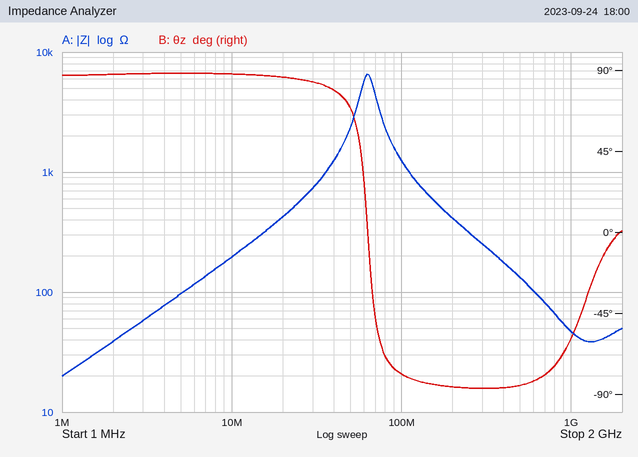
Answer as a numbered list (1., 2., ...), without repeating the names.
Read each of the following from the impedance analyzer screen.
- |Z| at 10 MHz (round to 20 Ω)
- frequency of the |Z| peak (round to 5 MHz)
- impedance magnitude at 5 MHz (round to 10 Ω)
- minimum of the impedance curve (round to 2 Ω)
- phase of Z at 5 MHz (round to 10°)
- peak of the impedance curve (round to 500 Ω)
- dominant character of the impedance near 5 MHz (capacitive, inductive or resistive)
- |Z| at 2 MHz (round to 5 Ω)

1. 200 Ω
2. 65 MHz
3. 100 Ω
4. 20 Ω
5. 90°
6. 6.5 kΩ
7. inductive
8. 40 Ω
